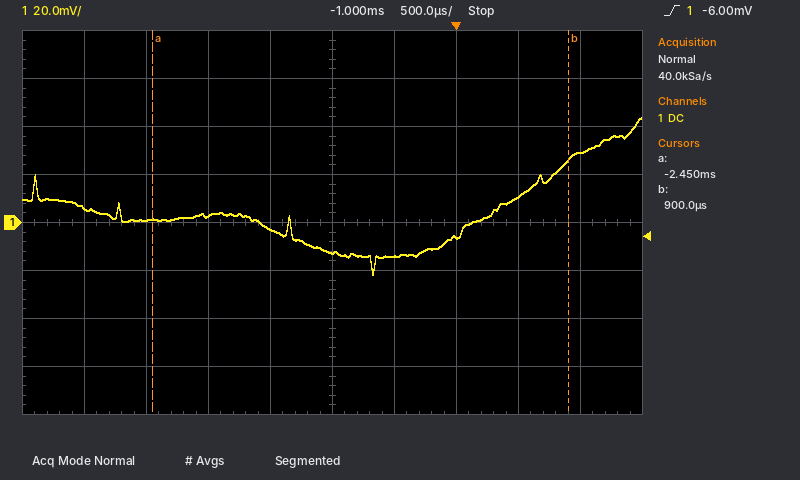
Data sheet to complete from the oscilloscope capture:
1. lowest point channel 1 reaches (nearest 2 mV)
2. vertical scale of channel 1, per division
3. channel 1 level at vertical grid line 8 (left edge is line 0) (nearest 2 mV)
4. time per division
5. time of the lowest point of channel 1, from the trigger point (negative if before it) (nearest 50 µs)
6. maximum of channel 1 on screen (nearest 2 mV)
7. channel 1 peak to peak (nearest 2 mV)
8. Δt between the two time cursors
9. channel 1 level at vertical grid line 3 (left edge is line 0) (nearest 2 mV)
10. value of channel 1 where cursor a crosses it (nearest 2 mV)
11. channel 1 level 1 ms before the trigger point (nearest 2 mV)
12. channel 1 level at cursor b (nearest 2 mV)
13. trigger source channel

-22 mV
20 mV
10 mV
500 µs
-650 µs
44 mV
66 mV
3.35 ms
2 mV
2 mV
-12 mV
26 mV
channel 1
